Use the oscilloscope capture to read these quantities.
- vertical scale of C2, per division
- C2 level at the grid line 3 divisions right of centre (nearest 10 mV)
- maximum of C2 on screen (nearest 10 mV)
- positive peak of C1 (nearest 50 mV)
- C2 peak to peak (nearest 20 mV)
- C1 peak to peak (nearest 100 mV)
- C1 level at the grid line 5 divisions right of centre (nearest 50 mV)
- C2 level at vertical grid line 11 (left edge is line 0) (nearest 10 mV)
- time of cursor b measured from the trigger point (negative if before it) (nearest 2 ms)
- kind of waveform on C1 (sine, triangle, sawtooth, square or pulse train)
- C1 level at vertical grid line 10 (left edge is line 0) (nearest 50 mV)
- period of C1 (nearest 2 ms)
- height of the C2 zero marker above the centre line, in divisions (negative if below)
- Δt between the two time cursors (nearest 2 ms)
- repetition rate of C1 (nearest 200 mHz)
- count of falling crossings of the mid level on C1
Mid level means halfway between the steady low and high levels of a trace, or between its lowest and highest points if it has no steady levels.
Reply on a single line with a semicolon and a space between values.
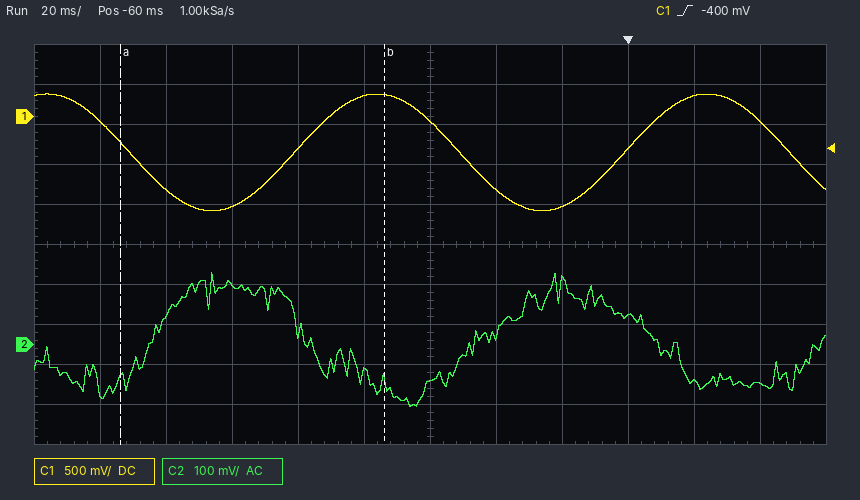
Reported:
100 mV; 70 mV; 180 mV; 300 mV; 340 mV; 1.50 V; -50 mV; -100 mV; -74 ms; sine; 250 mV; 100 ms; -2.5 div; 80 ms; 10.0 Hz; 3
